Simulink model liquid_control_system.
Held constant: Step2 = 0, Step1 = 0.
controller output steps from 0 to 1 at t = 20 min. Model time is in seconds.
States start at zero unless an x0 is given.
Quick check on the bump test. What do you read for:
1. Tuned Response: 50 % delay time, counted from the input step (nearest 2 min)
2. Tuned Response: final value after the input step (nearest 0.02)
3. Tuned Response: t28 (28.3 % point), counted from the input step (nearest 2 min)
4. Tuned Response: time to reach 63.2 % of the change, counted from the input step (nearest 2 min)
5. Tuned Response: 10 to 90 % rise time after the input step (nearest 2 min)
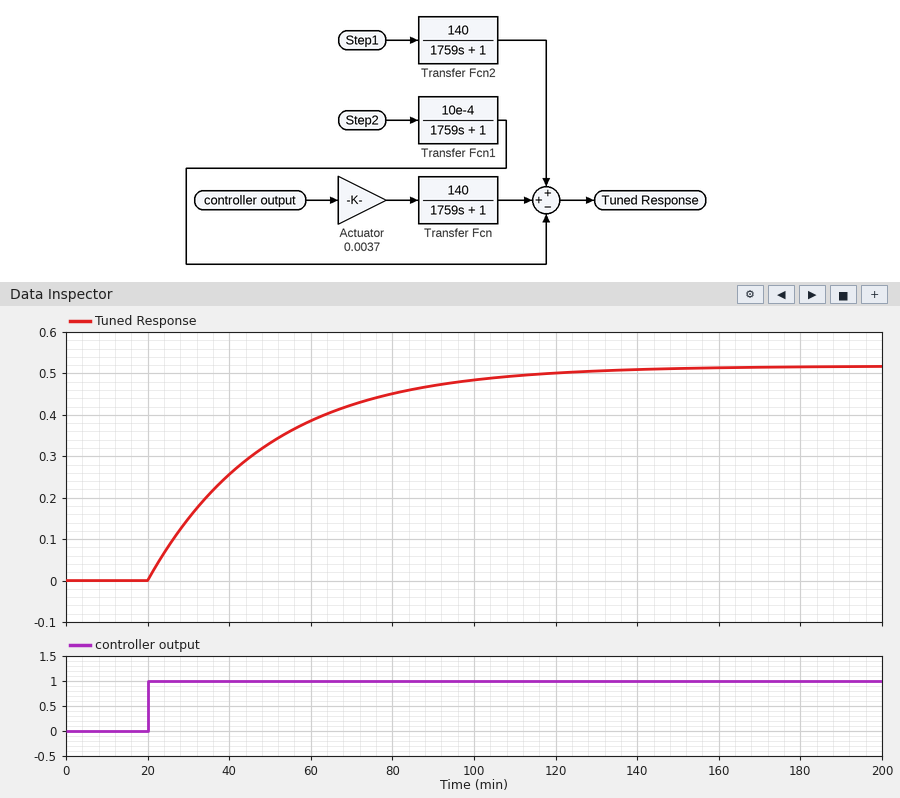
20 min
0.52
10 min
30 min
64 min
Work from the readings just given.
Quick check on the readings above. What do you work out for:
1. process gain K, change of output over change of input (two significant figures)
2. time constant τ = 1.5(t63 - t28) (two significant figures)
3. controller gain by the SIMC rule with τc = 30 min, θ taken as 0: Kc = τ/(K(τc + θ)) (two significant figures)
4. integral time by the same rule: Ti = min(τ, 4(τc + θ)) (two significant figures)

0.52
30 min
1.9
30 min
